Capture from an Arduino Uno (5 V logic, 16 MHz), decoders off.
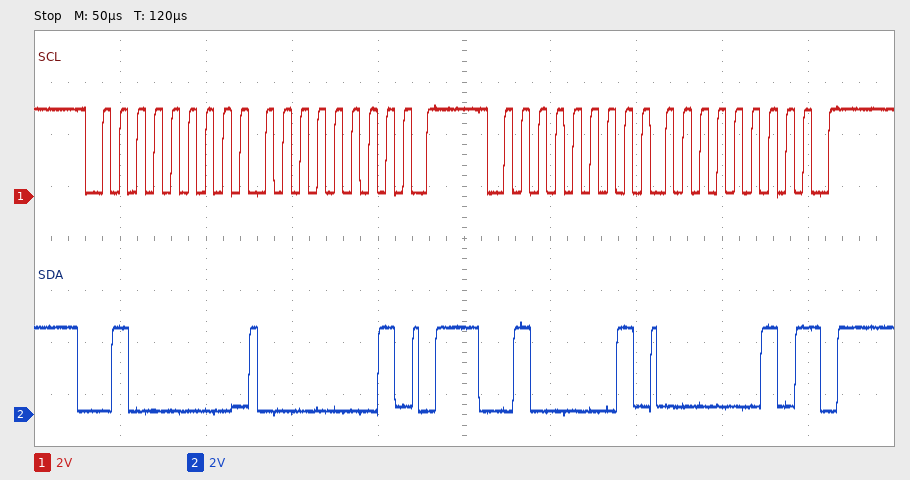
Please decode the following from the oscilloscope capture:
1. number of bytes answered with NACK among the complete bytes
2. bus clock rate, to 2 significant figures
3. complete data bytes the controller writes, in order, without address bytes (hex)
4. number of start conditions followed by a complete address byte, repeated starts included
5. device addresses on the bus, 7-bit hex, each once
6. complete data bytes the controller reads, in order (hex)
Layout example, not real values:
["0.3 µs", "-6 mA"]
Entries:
["1", "100 kHz", "01", "2", "0x20", "02"]
